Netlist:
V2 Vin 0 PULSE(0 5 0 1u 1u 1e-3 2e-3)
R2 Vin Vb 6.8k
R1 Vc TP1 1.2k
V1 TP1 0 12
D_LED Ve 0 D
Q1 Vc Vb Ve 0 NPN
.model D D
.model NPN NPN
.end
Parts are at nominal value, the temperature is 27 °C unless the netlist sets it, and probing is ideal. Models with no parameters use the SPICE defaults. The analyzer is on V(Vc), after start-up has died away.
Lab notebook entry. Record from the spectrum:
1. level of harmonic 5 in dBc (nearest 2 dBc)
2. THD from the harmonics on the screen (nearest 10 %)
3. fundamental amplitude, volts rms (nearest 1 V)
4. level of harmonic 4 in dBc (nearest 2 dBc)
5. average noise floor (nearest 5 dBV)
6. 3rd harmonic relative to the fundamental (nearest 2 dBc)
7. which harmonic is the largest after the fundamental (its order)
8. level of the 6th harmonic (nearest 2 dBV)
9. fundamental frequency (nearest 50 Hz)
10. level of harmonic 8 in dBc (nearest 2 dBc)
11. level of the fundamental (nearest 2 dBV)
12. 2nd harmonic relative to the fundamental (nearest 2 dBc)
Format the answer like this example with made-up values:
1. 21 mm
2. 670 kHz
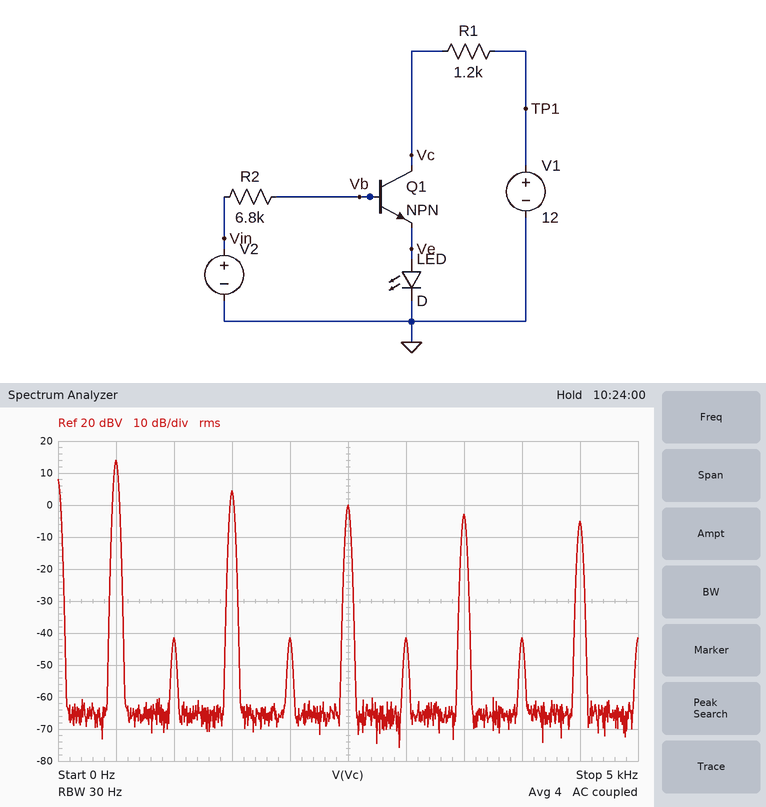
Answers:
1. -14 dBc
2. 40 %
3. 5 V
4. -56 dBc
5. -65 dBV
6. -10 dBc
7. 3
8. -42 dBV
9. 500 Hz
10. -56 dBc
11. 14 dBV
12. -56 dBc
